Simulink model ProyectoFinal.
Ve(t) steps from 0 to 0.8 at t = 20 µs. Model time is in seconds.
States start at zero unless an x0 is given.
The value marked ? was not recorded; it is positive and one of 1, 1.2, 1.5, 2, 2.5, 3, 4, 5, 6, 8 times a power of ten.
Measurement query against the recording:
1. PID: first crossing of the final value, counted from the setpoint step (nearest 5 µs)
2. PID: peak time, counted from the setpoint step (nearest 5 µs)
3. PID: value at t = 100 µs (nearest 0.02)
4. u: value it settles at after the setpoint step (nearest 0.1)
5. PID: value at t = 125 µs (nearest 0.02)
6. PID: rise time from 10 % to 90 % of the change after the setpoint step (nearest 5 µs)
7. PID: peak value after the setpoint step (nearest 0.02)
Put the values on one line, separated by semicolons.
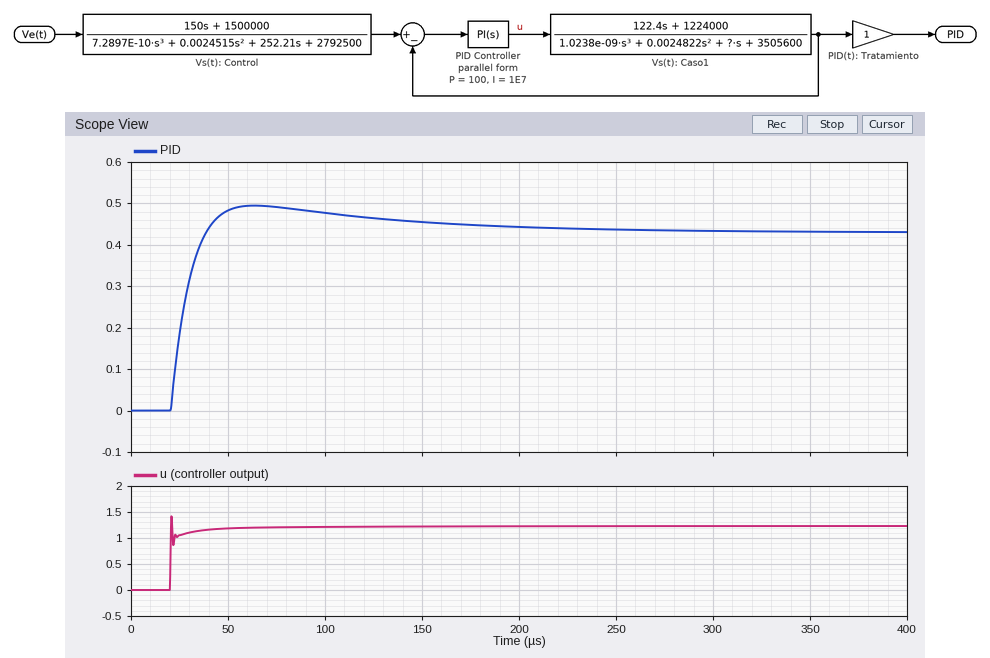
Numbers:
20 µs; 45 µs; 0.48; 1.2; 0.46; 15 µs; 0.50
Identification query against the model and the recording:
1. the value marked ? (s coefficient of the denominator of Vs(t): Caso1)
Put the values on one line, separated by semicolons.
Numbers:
300
